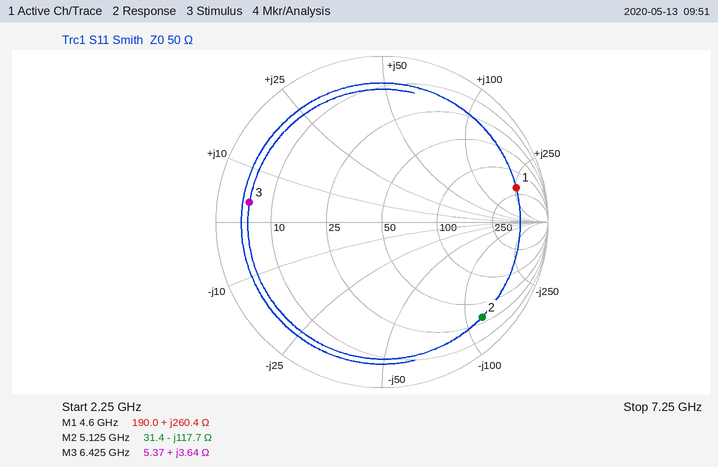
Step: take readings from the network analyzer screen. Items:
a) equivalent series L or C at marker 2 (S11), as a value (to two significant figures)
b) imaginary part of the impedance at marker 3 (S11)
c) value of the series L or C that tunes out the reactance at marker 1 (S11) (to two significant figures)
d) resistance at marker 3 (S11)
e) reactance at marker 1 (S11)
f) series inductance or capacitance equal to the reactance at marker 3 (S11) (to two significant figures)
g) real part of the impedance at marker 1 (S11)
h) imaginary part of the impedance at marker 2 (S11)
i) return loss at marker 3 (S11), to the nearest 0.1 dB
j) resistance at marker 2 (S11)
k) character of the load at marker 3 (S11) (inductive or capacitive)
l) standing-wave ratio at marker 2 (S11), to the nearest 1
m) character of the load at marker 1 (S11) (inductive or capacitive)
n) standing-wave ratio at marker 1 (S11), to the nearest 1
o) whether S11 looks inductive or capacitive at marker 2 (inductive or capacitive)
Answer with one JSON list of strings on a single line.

["260 fF", "+3.64 Ω", "130 fF", "5.37 Ω", "+260.4 Ω", "90 pH", "190.0 Ω", "-117.7 Ω", "1.9 dB", "31.4 Ω", "inductive", "11", "inductive", "11", "capacitive"]
